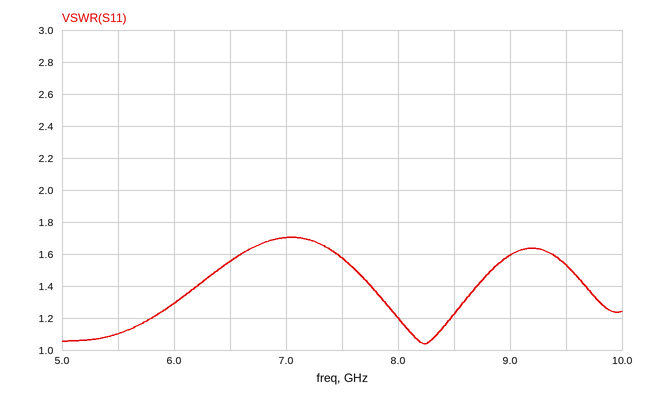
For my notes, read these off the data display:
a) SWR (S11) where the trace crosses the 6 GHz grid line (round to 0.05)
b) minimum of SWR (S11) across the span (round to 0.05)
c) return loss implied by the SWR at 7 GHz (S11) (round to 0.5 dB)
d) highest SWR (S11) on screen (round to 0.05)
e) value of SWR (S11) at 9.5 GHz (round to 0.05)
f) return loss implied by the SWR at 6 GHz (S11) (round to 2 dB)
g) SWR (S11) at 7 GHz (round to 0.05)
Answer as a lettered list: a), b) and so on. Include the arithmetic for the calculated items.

a) 1.30
b) 1.05
c) −20 log10((1.7 − 1)/(1.7 + 1)) ≈ 11.7 dB, so 11.5 dB to the nearest 0.5 dB
d) 1.70
e) 1.55
f) −20 log10((1.3 − 1)/(1.3 + 1)) ≈ 18 dB
g) 1.70
